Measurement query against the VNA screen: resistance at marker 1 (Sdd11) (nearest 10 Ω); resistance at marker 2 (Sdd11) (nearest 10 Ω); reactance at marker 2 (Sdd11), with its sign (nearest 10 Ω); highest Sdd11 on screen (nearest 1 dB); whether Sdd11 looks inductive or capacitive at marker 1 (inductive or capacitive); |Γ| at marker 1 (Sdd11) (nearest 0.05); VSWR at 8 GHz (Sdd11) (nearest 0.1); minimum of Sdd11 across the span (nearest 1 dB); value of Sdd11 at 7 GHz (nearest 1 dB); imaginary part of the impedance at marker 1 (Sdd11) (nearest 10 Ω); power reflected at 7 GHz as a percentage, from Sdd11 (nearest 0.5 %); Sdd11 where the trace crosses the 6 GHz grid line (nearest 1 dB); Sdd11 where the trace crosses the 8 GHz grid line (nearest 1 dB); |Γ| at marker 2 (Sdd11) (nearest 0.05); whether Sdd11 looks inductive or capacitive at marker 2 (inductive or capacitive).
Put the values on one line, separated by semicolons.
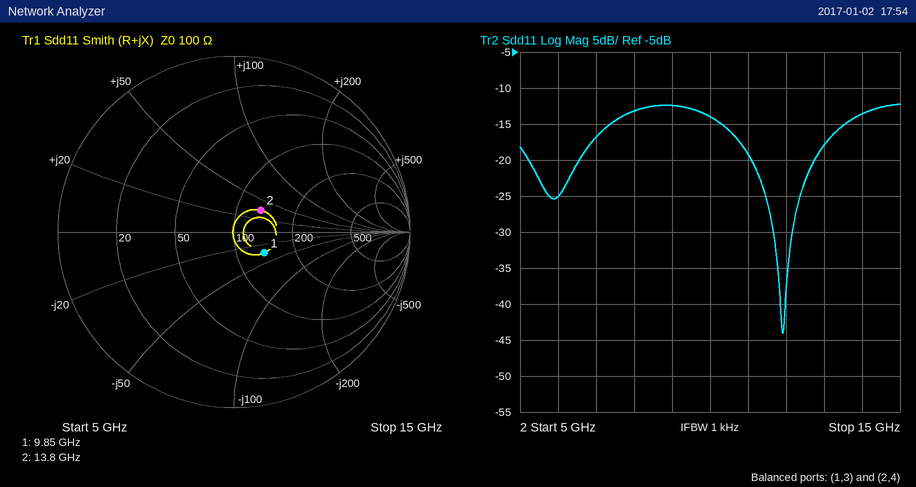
140 Ω; 130 Ω; +30 Ω; -12 dB; capacitive; 0.20; 1.6; -44 dB; -17 dB; -30 Ω; 2.0 %; -25 dB; -13 dB; 0.20; inductive
